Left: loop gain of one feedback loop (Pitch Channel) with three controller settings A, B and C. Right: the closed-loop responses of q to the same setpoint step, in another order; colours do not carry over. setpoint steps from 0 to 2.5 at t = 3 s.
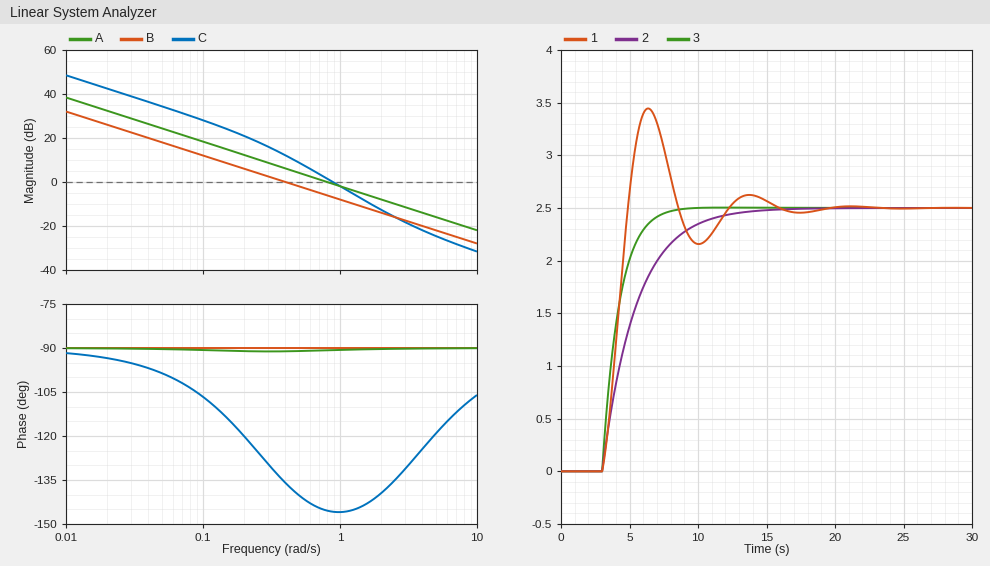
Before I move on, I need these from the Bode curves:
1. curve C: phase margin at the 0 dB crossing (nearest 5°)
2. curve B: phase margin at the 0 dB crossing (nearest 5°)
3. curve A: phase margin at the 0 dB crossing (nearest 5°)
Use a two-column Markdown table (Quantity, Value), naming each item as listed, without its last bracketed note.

| Quantity | Value |
|---|---|
| curve C: phase margin at the 0 dB crossing | 35° |
| curve B: phase margin at the 0 dB crossing | 90° |
| curve A: phase margin at the 0 dB crossing | 90° |
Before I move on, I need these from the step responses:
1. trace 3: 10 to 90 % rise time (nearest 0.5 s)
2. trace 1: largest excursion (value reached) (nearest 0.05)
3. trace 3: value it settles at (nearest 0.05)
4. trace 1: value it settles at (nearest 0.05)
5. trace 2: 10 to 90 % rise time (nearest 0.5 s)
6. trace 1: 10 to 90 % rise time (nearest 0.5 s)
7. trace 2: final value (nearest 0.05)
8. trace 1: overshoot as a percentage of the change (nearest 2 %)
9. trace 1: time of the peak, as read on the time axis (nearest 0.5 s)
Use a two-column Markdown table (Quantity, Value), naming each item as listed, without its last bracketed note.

| Quantity | Value |
|---|---|
| trace 3: 10 to 90 % rise time | 2.5 s |
| trace 1: largest excursion (value reached) | 3.45 |
| trace 3: value it settles at | 2.50 |
| trace 1: value it settles at | 2.50 |
| trace 2: 10 to 90 % rise time | 5.5 s |
| trace 1: 10 to 90 % rise time | 1.5 s |
| trace 2: final value | 2.50 |
| trace 1: overshoot as a percentage of the change | 38 % |
| trace 1: time of the peak, as read on the time axis | 6.5 s |
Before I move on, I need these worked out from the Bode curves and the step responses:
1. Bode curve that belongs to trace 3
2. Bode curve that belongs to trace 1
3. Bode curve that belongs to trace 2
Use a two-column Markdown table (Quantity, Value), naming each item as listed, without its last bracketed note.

| Quantity | Value |
|---|---|
| Bode curve that belongs to trace 3 | A |
| Bode curve that belongs to trace 1 | C |
| Bode curve that belongs to trace 2 | B |
